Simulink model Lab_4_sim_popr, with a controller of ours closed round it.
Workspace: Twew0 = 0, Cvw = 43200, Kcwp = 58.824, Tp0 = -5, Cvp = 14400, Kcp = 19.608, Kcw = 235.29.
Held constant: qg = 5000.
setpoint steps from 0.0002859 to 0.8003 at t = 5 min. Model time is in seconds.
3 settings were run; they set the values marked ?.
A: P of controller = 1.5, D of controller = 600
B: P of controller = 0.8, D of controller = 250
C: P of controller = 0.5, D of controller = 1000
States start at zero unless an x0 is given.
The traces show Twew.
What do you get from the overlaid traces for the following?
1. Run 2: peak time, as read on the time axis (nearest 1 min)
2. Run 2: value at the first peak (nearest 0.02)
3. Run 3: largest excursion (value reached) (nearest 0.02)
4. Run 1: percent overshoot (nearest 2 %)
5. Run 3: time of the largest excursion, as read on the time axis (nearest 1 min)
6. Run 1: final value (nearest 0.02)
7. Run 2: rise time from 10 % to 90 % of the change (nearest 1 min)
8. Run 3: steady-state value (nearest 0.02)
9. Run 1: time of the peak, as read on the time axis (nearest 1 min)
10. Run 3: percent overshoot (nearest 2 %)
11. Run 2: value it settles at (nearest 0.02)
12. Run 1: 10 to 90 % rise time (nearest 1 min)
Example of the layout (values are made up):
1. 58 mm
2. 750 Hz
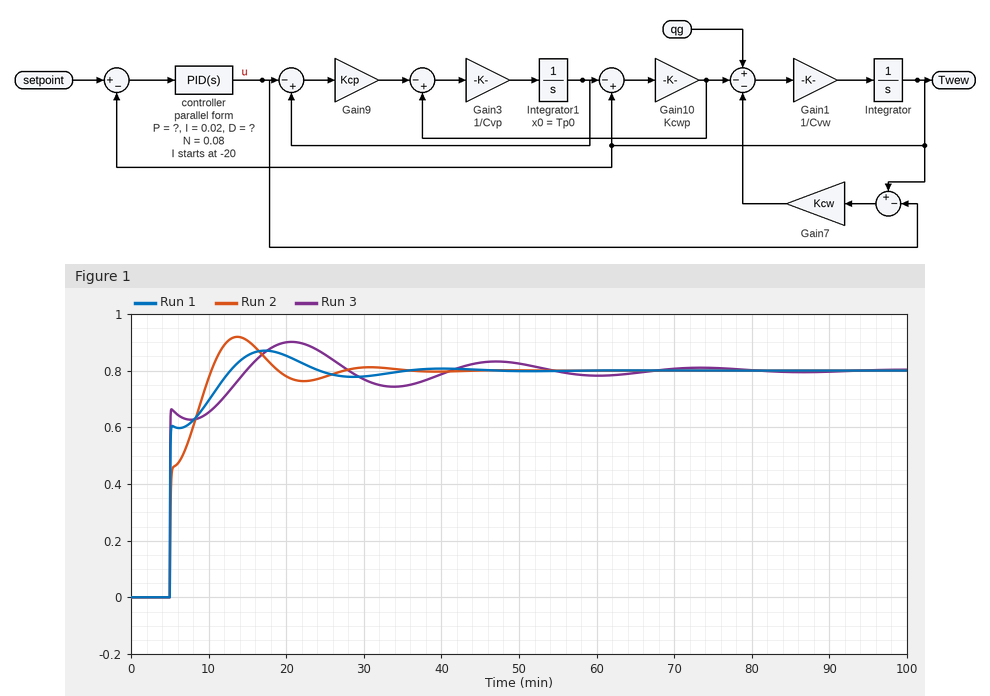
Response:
1. 14 min
2. 0.92
3. 0.90
4. 8 %
5. 21 min
6. 0.80
7. 4 min
8. 0.80
9. 17 min
10. 12 %
11. 0.80
12. 6 min
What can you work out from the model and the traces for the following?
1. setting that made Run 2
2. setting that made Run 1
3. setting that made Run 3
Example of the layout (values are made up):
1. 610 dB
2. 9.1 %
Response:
1. B
2. A
3. C
